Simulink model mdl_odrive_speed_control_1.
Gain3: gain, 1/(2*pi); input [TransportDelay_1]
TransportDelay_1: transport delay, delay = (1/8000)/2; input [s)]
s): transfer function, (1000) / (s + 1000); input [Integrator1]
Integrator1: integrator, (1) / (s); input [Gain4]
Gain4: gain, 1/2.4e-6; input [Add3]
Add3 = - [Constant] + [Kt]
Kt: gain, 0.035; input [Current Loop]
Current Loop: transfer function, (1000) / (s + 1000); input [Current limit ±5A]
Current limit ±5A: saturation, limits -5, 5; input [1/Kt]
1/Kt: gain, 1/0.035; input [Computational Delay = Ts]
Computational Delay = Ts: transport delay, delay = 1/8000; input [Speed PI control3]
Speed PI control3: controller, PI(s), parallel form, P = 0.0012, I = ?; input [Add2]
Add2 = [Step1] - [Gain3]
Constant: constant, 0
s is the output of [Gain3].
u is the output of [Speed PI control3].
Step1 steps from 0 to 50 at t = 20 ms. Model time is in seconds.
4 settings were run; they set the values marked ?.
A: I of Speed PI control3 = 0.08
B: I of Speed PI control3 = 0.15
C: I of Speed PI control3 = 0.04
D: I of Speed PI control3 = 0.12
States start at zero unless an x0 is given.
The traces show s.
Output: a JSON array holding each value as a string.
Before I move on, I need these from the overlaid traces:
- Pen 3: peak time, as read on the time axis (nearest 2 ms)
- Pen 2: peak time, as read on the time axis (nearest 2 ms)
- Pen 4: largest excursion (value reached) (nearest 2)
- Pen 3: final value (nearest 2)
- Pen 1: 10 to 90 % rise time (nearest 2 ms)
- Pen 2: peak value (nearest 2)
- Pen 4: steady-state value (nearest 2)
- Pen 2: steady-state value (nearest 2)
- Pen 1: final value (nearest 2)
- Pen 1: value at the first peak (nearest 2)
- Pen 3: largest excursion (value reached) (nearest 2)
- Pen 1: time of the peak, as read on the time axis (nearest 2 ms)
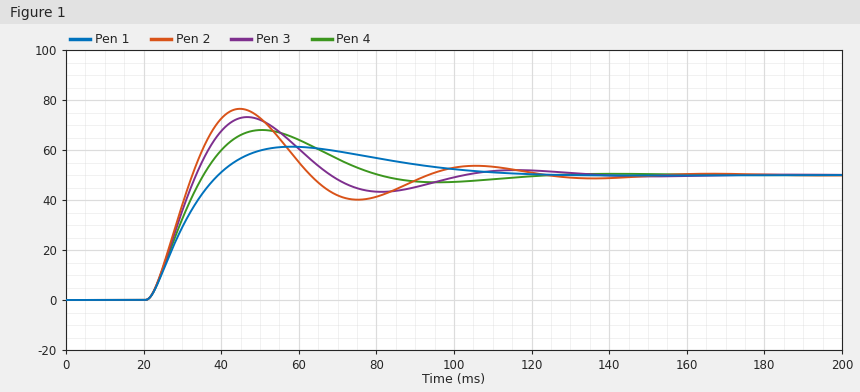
["46 ms", "44 ms", "68", "50", "14 ms", "76", "50", "50", "50", "62", "74", "58 ms"]
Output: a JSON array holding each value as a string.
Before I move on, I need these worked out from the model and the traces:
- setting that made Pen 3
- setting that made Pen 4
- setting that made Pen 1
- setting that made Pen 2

["D", "A", "C", "B"]
